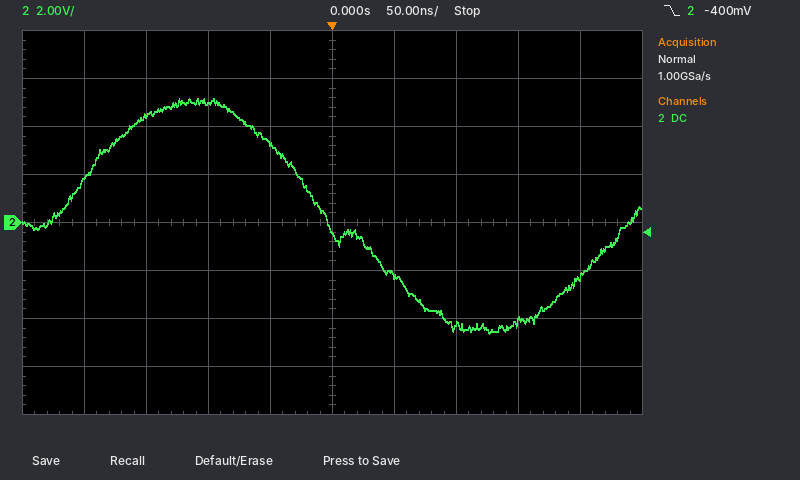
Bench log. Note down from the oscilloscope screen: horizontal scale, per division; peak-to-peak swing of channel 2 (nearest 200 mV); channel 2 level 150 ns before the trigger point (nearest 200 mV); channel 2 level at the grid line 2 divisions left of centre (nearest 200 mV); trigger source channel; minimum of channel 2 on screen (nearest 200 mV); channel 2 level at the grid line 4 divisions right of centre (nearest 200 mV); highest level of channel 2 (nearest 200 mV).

50 ns
9.8 V
4.4 V
5.0 V
channel 2
-4.6 V
-2.2 V
5.2 V
